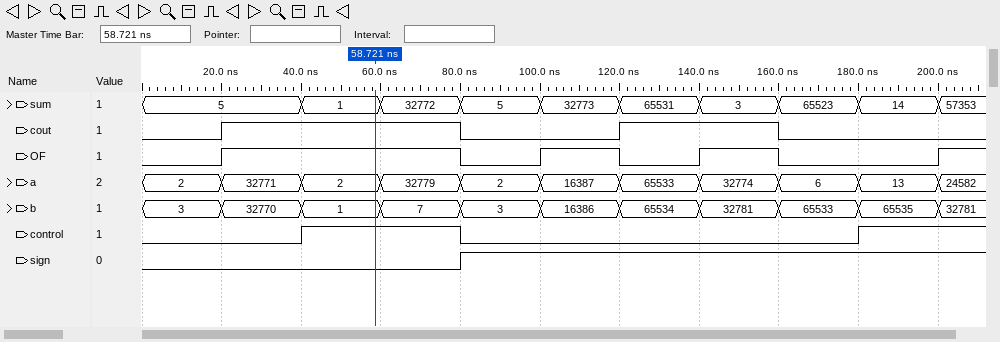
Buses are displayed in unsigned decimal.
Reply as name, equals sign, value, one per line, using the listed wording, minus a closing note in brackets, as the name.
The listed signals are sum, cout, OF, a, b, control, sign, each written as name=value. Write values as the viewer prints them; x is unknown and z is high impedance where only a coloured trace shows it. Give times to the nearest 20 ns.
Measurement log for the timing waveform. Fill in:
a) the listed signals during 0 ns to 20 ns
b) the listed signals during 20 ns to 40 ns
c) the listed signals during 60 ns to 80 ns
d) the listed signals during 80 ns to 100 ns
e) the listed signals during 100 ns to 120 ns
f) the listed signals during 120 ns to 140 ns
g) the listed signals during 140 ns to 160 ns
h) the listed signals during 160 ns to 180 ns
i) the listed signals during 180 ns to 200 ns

the listed signals during 0 ns to 20 ns = sum=5, cout=0, OF=0, a=2, b=3, control=0, sign=0
the listed signals during 20 ns to 40 ns = sum=5, cout=1, OF=1, a=32771, b=32770, control=0, sign=0
the listed signals during 60 ns to 80 ns = sum=32772, cout=1, OF=1, a=32779, b=7, control=1, sign=0
the listed signals during 80 ns to 100 ns = sum=5, cout=0, OF=0, a=2, b=3, control=0, sign=1
the listed signals during 100 ns to 120 ns = sum=32773, cout=0, OF=1, a=16387, b=16386, control=0, sign=1
the listed signals during 120 ns to 140 ns = sum=65531, cout=1, OF=0, a=65533, b=65534, control=0, sign=1
the listed signals during 140 ns to 160 ns = sum=3, cout=1, OF=1, a=32774, b=32781, control=0, sign=1
the listed signals during 160 ns to 180 ns = sum=65523, cout=0, OF=0, a=6, b=65533, control=0, sign=1
the listed signals during 180 ns to 200 ns = sum=14, cout=0, OF=0, a=13, b=65535, control=1, sign=1
